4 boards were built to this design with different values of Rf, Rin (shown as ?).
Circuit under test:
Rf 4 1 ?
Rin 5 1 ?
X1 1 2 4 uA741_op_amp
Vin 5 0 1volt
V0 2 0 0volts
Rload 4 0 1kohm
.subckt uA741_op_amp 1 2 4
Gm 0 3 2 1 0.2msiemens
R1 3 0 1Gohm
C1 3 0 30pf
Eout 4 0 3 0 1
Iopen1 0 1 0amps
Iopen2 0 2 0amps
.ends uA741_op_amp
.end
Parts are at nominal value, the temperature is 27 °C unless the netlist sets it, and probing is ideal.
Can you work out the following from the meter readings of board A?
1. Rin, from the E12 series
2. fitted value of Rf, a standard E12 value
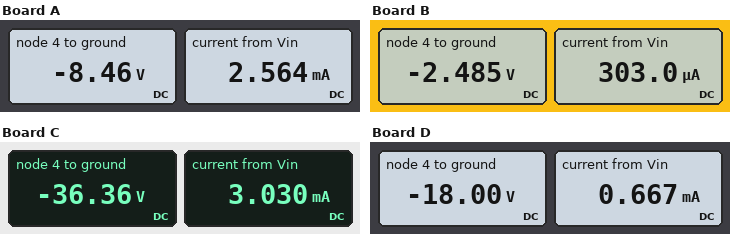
390 Ω
3.3 kΩ
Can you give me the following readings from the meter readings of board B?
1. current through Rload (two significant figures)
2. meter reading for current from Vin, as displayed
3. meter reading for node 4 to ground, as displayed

2.5 mA
303.0 µA
-2.485 V
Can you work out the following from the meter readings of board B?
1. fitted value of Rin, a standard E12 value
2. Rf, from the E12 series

3.3 kΩ
8.2 kΩ
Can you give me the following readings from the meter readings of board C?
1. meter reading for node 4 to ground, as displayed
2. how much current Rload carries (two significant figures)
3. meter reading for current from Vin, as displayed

-36.36 V
36 mA
3.030 mA
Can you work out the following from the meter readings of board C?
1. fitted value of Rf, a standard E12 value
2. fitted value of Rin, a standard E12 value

12 kΩ
330 Ω
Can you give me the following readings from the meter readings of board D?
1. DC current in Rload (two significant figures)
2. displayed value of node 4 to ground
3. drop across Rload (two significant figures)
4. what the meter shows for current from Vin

18 mA
-18.00 V
18 V
0.667 mA
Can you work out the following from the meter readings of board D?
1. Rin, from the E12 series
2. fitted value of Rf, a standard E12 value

1.5 kΩ
27 kΩ
